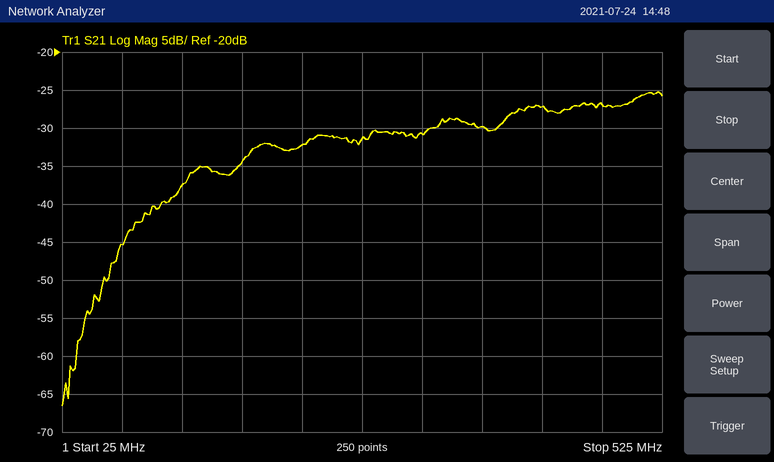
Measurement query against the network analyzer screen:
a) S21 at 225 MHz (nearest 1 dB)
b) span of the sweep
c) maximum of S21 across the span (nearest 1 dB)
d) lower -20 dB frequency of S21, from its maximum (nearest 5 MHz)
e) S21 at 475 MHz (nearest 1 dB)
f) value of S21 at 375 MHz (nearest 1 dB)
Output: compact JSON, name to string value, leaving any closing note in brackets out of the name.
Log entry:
{"S21 at 225 MHz": "-32 dB", "span of the sweep": "500 MHz", "maximum of S21 across the span": "-25 dB", "lower -20 dB frequency of S21, from its maximum": "75 MHz", "S21 at 475 MHz": "-27 dB", "value of S21 at 375 MHz": "-30 dB"}
